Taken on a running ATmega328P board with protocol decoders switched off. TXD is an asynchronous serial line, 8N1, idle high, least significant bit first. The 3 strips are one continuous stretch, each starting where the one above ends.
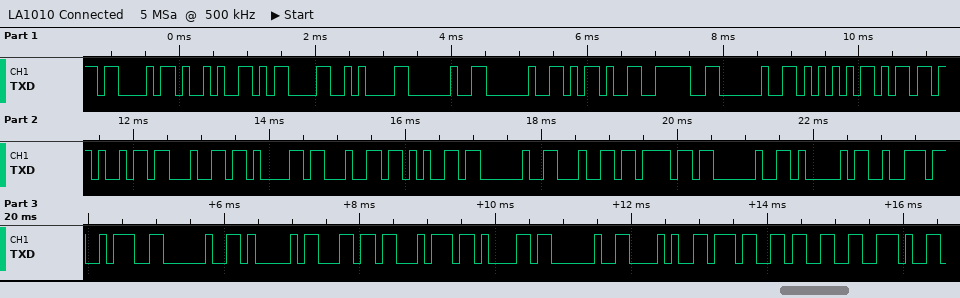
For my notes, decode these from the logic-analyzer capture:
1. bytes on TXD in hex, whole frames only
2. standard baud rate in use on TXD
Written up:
0x43 0x29 0x0D 0x0A 0x20 0x20 0x2D 0x3E 0x20 0x55 0x6D 0x69 0x64 0x61 0x64 0x65 0x20 0x64 0x6F 0x20 0x41 0x72 0x3A 0x20 0x41 0x6C 0x74 0x61 0x20 0x28 0x37 0x33 0x2E
9600 baud
